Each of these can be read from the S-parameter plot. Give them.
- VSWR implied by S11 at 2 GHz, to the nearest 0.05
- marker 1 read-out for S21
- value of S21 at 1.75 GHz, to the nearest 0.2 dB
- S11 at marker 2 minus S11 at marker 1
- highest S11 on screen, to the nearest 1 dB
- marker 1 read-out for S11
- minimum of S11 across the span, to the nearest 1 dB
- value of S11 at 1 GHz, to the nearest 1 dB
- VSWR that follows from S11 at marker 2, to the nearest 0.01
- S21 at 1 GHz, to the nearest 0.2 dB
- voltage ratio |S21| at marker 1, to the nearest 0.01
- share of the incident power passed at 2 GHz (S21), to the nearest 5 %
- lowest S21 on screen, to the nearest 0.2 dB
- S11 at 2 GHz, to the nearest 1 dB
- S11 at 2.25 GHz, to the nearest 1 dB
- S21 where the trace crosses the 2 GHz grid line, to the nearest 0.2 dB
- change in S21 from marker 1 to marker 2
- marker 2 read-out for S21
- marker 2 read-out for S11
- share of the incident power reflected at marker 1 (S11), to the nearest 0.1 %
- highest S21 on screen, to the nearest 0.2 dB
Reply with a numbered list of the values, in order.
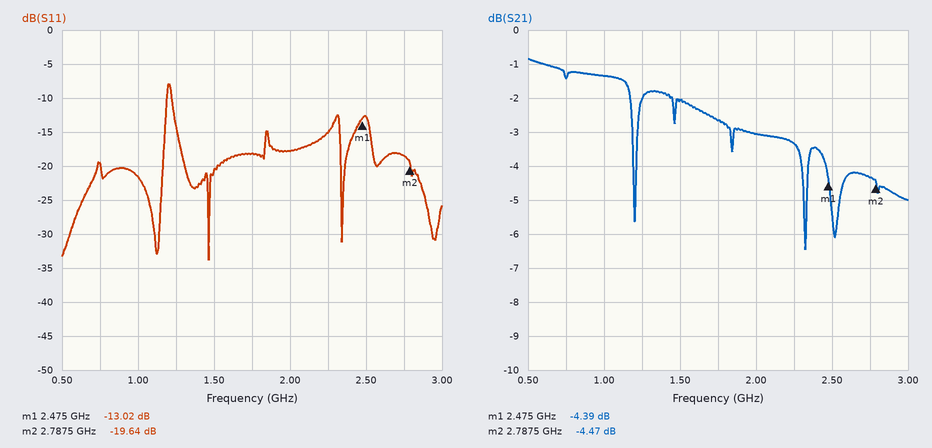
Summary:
1. 1.30
2. -4.39 dB
3. -2.6 dB
4. -6.62 dB
5. -8 dB
6. -13.02 dB
7. -34 dB
8. -22 dB
9. 1.23
10. -1.4 dB
11. 0.60
12. 50 %
13. -6.4 dB
14. -18 dB
15. -15 dB
16. -3.0 dB
17. -0.08 dB
18. -4.47 dB
19. -19.64 dB
20. 5.0 %
21. -0.8 dB
